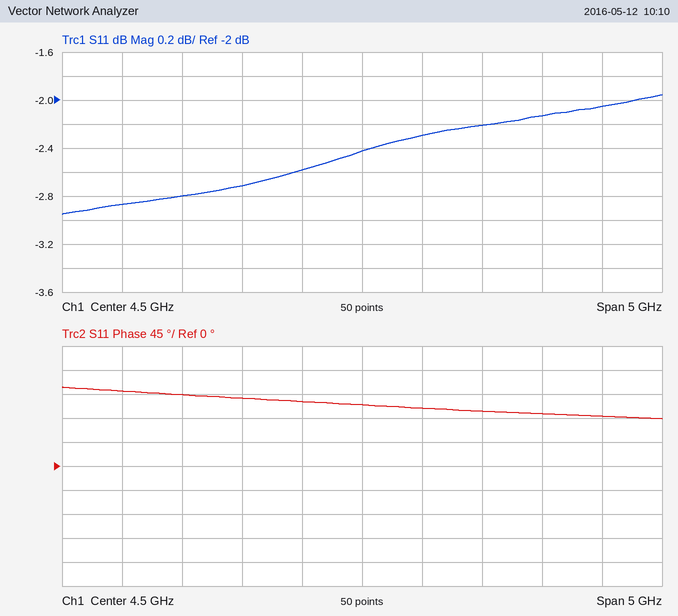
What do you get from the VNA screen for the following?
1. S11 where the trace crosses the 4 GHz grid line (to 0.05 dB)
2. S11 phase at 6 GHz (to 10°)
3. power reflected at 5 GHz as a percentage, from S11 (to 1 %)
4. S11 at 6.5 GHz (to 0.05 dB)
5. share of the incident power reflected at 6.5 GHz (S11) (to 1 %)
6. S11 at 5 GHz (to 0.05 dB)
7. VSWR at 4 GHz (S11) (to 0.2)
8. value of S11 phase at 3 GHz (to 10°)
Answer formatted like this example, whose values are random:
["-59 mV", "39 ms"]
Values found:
["-2.60 dB", "100°", "59 %", "-2.05 dB", "62 %", "-2.30 dB", "6.8", "130°"]
